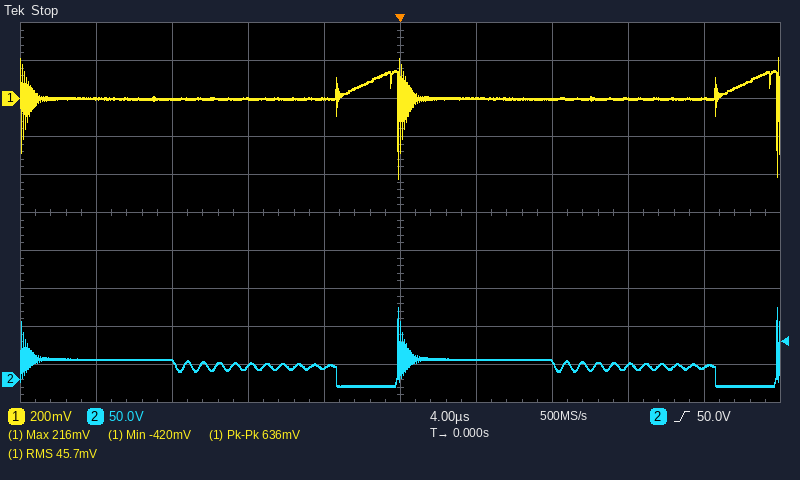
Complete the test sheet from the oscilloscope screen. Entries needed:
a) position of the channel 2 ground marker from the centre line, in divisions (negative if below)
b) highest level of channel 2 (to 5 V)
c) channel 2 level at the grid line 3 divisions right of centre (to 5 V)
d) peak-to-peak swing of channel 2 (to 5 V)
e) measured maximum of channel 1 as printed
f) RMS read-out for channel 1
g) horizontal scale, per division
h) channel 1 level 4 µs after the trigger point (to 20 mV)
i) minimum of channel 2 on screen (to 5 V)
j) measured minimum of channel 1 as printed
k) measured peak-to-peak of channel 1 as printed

-4.4 div
95 V
20 V
105 V
216 mV
45.7 mV
4 µs
0 mV
-10 V
-420 mV
636 mV
